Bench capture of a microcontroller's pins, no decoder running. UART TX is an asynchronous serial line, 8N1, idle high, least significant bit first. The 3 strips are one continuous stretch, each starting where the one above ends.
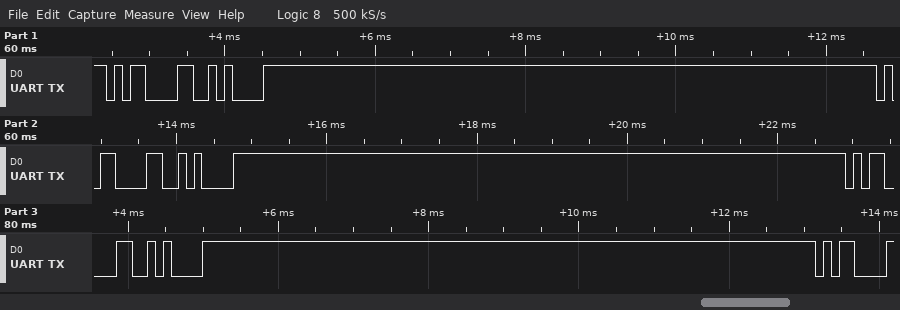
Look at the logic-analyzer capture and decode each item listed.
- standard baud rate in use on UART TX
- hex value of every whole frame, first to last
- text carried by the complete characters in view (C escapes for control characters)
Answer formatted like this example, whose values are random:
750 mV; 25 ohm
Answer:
9600 baud; 0x0D 0x0A 0x0D 0x0A 0x0D 0x0A 0x0D; "\r\n\r\n\r\n\r"
